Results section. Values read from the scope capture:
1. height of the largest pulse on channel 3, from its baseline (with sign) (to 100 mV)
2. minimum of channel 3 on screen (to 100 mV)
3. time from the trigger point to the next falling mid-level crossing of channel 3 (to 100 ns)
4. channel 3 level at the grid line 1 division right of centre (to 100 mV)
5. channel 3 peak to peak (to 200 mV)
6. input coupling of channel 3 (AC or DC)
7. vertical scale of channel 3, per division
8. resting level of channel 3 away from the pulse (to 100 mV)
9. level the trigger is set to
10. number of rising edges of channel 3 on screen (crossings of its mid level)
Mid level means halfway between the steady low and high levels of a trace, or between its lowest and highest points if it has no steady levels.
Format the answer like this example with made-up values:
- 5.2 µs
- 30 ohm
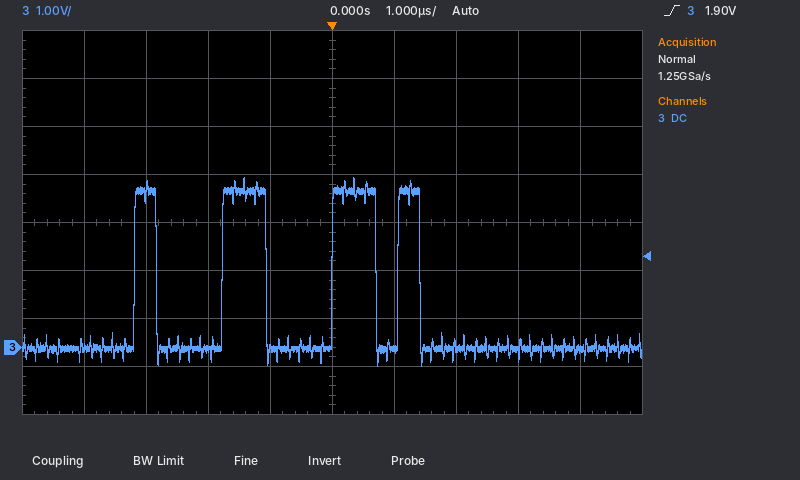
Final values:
- +3.6 V
- -400 mV
- 700 ns
- 0.0 V
- 4.0 V
- DC
- 1 V
- 0.0 V
- 1.90 V
- 4
